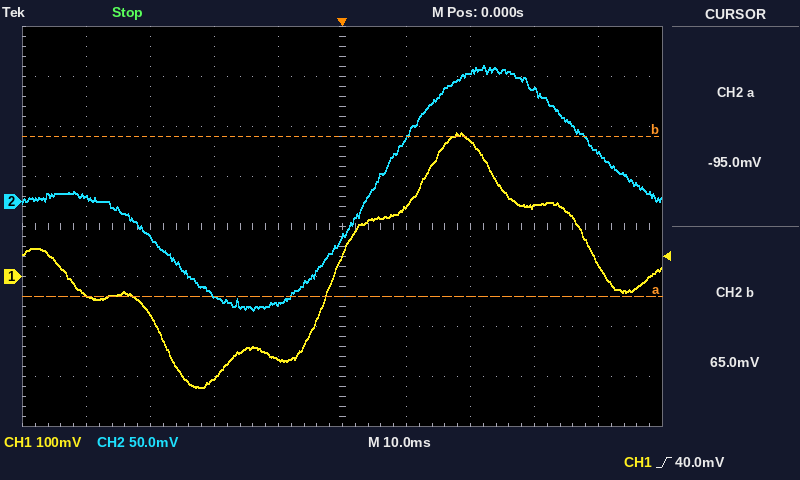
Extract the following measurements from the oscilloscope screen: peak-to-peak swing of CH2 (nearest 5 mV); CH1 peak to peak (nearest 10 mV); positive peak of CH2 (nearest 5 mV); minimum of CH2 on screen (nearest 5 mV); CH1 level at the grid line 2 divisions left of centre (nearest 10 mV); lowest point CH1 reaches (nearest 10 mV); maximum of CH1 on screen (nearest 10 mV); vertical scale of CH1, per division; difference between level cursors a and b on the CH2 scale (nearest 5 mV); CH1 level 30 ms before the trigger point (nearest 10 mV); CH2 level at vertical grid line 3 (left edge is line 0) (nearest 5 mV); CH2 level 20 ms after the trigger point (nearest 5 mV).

245 mV
510 mV
135 mV
-110 mV
-200 mV
-220 mV
290 mV
100 mV
160 mV
-80 mV
-95 mV
130 mV
